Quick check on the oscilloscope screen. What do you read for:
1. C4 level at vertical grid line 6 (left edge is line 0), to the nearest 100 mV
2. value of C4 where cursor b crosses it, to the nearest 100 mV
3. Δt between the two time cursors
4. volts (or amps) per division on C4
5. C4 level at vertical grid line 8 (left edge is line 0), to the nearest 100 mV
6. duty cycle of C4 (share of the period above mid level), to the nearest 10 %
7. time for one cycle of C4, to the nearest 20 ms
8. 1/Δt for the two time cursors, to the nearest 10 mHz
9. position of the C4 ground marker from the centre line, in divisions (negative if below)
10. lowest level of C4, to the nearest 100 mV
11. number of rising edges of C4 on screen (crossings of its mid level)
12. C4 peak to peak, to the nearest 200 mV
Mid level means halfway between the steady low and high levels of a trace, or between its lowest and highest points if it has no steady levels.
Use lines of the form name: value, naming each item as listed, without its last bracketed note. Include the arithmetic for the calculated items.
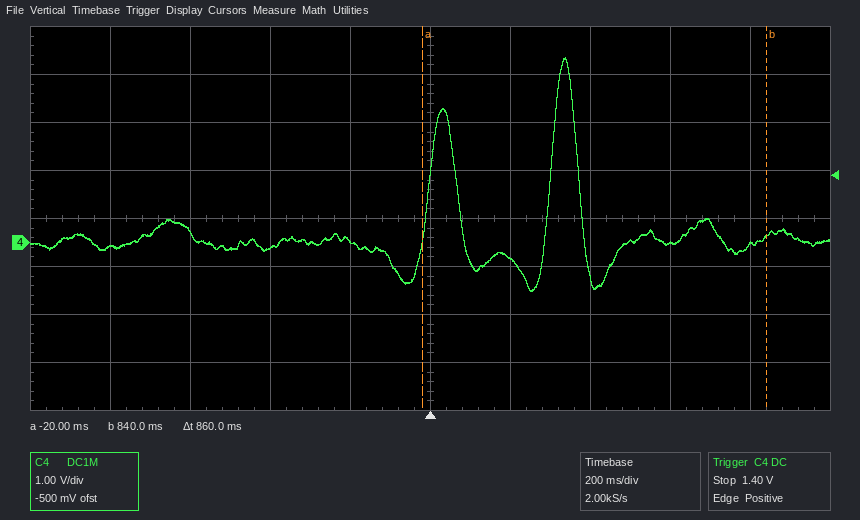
C4 level at vertical grid line 6 (left edge is line 0), to the nearest 100 mV: -300 mV
value of C4 where cursor b crosses it, to the nearest 100 mV: 100 mV
Δt between the two time cursors: 860 ms
volts (or amps) per division on C4: 1 V
C4 level at vertical grid line 8 (left edge is line 0), to the nearest 100 mV: 0.0 V
duty cycle of C4 (share of the period above mid level), to the nearest 10 %: 20 %
time for one cycle of C4, to the nearest 20 ms: 300 ms
1/Δt for the two time cursors, to the nearest 10 mHz: 1 / 860 ms ≈ 1.16 Hz
position of the C4 ground marker from the centre line, in divisions: -0.5 div
lowest level of C4, to the nearest 100 mV: -1.0 V
number of rising edges of C4 on screen: 2
C4 peak to peak, to the nearest 200 mV: 4.8 V
